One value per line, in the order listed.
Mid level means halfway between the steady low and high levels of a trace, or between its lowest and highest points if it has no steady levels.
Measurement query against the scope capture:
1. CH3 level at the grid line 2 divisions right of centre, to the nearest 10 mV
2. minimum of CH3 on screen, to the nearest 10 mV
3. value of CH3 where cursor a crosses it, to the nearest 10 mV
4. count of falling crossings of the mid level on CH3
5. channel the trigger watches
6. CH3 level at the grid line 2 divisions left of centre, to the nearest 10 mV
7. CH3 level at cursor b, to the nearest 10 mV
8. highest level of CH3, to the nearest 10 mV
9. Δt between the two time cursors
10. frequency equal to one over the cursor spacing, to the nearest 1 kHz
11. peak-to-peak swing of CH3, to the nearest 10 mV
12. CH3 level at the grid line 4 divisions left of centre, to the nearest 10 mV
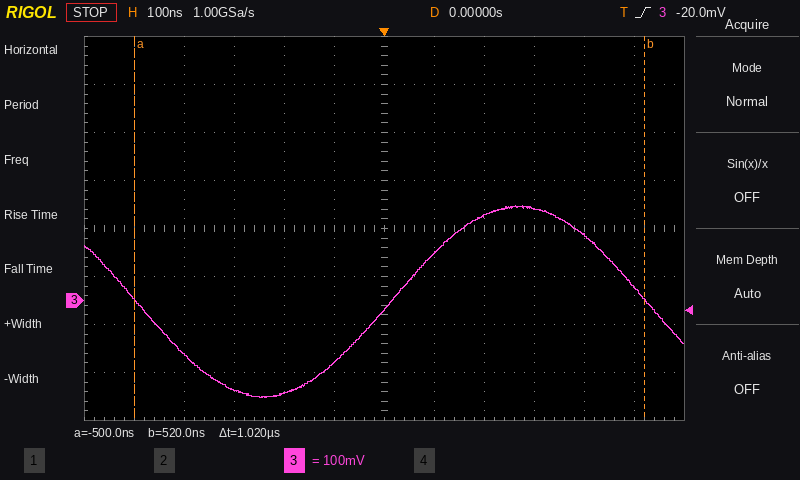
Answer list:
180 mV
-200 mV
0 mV
2
CH3
-190 mV
0 mV
200 mV
1.02 µs
980 kHz
400 mV
-110 mV
